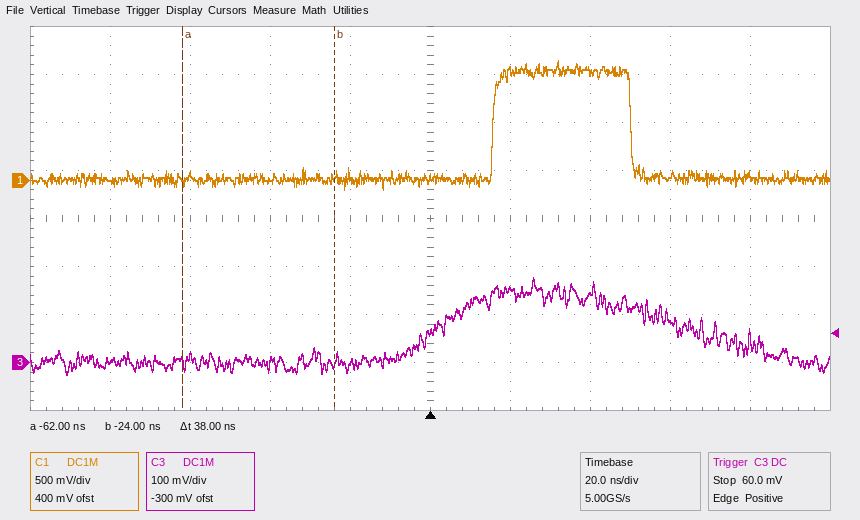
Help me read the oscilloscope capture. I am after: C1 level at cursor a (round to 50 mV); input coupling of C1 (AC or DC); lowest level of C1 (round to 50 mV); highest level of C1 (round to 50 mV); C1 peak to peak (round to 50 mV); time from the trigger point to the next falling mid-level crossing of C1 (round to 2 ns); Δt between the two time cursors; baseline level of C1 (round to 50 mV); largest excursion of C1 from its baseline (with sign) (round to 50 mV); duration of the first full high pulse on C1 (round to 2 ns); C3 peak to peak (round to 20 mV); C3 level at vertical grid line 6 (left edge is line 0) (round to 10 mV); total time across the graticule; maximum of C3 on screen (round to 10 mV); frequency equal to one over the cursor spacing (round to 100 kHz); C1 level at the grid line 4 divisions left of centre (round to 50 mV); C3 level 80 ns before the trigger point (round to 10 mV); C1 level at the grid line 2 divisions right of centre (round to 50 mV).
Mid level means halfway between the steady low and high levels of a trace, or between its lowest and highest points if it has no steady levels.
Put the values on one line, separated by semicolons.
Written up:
0 mV; DC; -100 mV; 1.25 V; 1.35 V; 50 ns; 38 ns; 0 mV; +1.25 V; 34 ns; 200 mV; 150 mV; 200 ns; 180 mV; 26.3 MHz; 0 mV; 0 mV; 1.15 V
